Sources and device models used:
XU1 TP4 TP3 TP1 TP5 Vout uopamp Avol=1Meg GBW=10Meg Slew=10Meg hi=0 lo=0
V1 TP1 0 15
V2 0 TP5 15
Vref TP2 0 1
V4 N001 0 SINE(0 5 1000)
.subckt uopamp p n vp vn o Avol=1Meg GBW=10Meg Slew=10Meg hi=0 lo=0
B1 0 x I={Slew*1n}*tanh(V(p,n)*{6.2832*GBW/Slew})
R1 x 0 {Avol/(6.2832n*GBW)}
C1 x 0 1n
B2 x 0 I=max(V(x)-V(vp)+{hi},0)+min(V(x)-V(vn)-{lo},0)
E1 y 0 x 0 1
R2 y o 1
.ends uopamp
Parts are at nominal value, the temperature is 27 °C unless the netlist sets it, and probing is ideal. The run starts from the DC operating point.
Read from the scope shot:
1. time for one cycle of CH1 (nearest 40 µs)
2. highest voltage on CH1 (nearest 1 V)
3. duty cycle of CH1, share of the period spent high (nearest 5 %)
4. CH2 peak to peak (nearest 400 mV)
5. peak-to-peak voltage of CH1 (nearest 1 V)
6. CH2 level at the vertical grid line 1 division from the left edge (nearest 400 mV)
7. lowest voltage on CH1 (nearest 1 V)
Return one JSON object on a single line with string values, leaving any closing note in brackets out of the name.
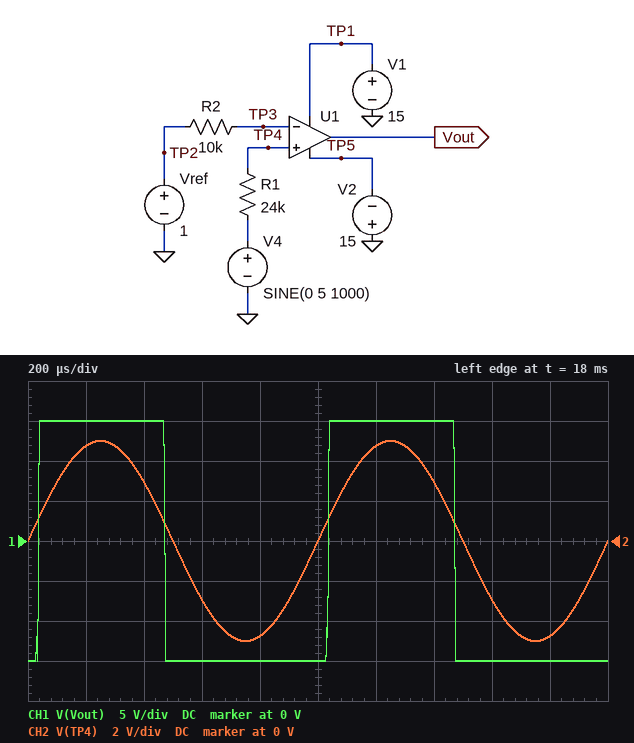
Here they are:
{"time for one cycle of CH1": "1.00 ms", "highest voltage on CH1": "15 V", "duty cycle of CH1, share of the period spent high": "45 %", "CH2 peak to peak": "10.0 V", "peak-to-peak voltage of CH1": "30 V", "CH2 level at the vertical grid line 1 division from the left edge": "4.8 V", "lowest voltage on CH1": "-15 V"}
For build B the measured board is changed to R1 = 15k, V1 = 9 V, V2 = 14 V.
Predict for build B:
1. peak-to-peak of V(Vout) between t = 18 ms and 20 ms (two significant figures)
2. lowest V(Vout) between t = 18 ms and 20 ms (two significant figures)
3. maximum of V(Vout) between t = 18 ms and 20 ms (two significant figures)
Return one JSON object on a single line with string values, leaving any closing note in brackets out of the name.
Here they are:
{"peak-to-peak of V(Vout) between t = 18 ms and 20 ms": "23 V", "lowest V(Vout) between t = 18 ms and 20 ms": "-14 V", "maximum of V(Vout) between t = 18 ms and 20 ms": "9.0 V"}
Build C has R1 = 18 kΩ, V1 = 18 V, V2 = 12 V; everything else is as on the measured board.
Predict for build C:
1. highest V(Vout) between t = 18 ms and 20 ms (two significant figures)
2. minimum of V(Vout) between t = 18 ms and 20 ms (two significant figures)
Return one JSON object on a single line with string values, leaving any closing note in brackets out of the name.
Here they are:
{"highest V(Vout) between t = 18 ms and 20 ms": "18 V", "minimum of V(Vout) between t = 18 ms and 20 ms": "-12 V"}
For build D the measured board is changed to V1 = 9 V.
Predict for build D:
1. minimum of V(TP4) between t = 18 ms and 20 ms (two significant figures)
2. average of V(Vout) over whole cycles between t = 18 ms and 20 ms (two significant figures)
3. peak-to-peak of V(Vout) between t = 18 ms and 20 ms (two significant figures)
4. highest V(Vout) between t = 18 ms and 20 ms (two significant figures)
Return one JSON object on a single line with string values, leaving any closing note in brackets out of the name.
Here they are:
{"minimum of V(TP4) between t = 18 ms and 20 ms": "-5.0 V", "average of V(Vout) over whole cycles between t = 18 ms and 20 ms": "-4.5 V", "peak-to-peak of V(Vout) between t = 18 ms and 20 ms": "24 V", "highest V(Vout) between t = 18 ms and 20 ms": "9.0 V"}
